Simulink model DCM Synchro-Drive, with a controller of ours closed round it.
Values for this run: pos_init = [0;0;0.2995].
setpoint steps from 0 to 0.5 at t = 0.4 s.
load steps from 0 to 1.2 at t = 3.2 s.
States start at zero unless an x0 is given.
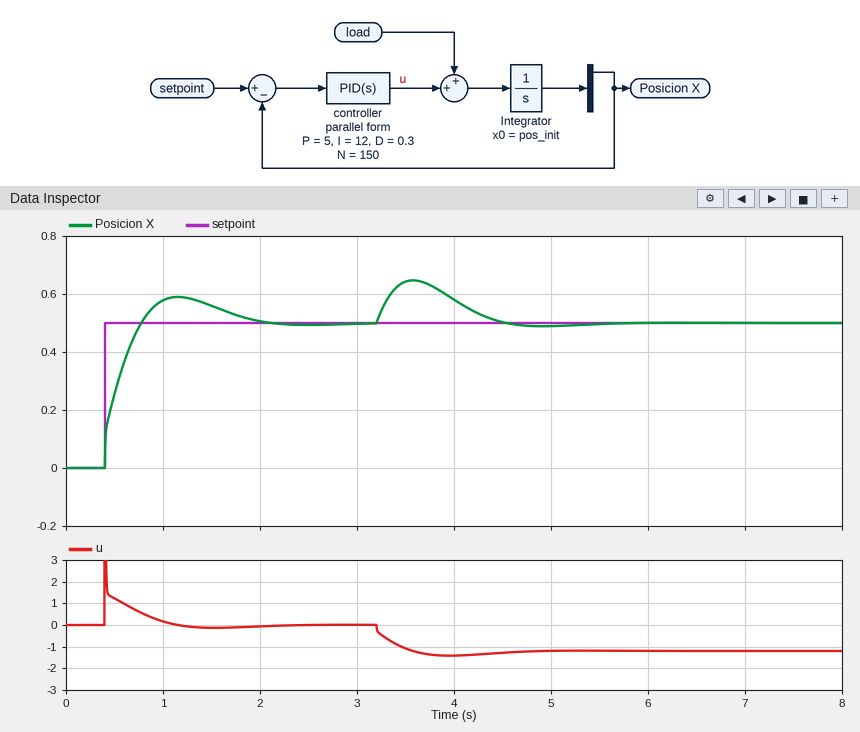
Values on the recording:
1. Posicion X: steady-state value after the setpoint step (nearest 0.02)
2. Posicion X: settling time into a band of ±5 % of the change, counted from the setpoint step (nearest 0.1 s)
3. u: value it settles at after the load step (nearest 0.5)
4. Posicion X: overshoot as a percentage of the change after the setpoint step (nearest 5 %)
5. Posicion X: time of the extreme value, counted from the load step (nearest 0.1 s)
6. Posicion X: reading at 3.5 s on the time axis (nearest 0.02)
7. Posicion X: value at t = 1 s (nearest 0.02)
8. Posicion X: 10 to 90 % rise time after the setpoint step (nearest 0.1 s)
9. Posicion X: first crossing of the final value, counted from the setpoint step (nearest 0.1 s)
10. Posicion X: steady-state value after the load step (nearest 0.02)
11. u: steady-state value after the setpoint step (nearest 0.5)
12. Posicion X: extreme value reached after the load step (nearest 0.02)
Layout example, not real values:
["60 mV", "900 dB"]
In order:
["0.50", "1.4 s", "-1.0", "20 %", "0.4 s", "0.64", "0.58", "0.3 s", "0.4 s", "0.50", "0.0", "0.64"]
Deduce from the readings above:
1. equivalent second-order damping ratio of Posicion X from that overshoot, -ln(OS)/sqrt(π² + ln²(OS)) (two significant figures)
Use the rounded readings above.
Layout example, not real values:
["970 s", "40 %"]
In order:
["0.46"]
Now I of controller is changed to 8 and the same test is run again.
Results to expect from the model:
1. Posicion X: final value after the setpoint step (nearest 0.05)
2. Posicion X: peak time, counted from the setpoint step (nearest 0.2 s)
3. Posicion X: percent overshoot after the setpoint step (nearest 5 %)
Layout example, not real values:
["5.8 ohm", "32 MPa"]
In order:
["0.50", "0.8 s", "15 %"]
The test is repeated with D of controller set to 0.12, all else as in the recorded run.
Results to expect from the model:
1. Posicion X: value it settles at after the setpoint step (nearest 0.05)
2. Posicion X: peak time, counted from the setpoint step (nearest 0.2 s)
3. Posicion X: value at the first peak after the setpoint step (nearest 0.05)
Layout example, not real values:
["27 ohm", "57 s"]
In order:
["0.50", "0.6 s", "0.60"]
